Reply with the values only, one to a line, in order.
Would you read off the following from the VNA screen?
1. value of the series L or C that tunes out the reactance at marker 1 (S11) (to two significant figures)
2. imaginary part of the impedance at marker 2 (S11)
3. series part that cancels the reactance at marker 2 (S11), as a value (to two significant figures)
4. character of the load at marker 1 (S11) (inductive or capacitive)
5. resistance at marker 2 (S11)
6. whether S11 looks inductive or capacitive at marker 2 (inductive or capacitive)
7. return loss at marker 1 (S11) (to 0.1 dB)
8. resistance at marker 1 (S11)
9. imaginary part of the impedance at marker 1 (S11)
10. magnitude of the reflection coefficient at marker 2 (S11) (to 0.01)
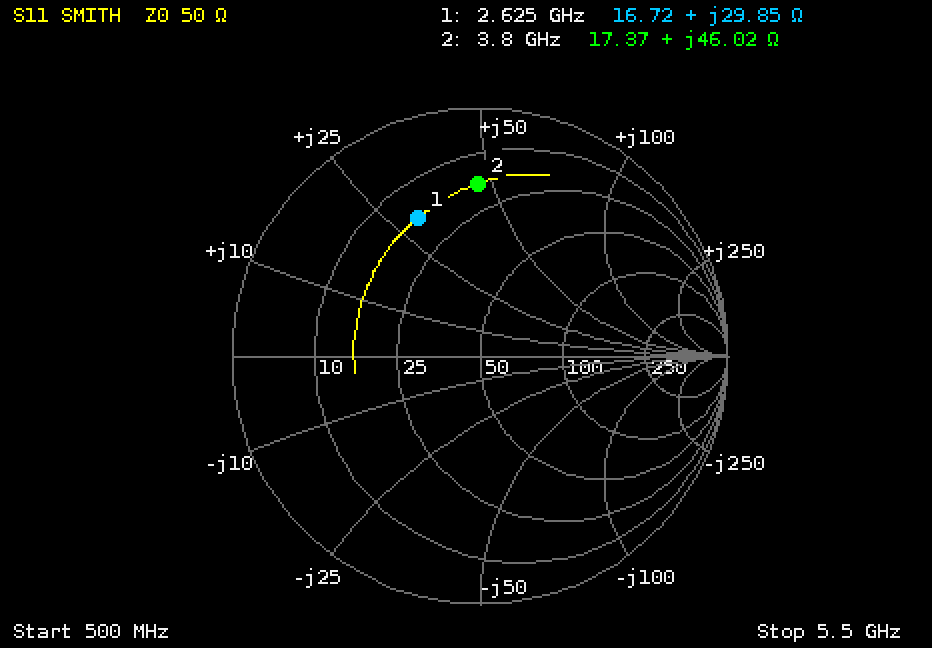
2.0 pF
+46.02 Ω
910 fF
inductive
17.37 Ω
inductive
4.3 dB
16.72 Ω
+29.85 Ω
0.69
